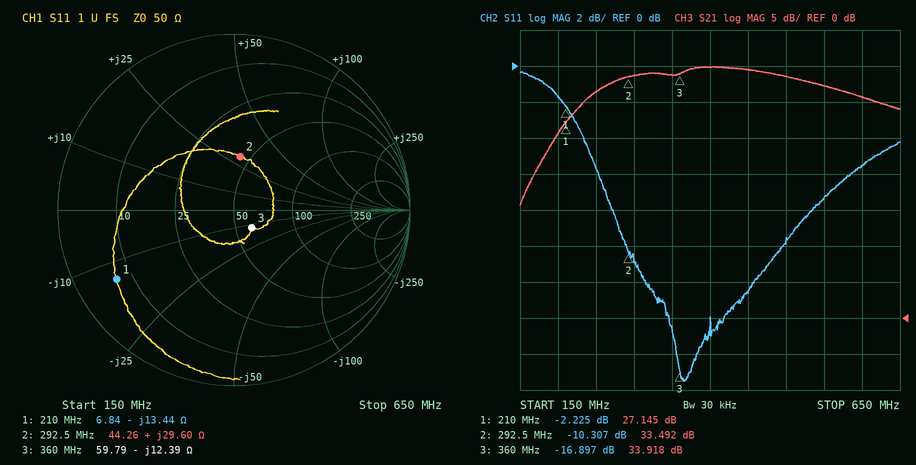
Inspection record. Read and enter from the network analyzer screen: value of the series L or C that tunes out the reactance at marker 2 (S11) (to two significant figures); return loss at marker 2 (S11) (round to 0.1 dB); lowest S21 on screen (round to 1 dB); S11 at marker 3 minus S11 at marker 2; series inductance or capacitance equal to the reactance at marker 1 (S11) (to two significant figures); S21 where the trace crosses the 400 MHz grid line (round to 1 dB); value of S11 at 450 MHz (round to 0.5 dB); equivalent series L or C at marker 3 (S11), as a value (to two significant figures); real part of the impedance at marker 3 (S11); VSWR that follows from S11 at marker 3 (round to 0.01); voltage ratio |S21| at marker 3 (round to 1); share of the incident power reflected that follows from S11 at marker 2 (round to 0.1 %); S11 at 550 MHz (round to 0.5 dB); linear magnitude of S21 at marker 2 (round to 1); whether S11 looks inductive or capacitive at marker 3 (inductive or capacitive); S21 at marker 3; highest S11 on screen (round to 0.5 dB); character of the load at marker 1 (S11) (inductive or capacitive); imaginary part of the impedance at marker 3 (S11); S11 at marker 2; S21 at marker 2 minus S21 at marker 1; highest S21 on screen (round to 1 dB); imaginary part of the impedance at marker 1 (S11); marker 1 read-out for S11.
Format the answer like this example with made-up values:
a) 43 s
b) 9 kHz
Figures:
a) 18 pF
b) 10.3 dB
c) 16 dB
d) -6.590 dB
e) 56 pF
f) 35 dB
g) -12.5 dB
h) 36 pF
i) 59.79 Ω
j) 1.33
k) 50
l) 9.3 %
m) -7.5 dB
n) 47
o) capacitive
p) 33.918 dB
q) -0.5 dB
r) capacitive
s) -12.39 Ω
t) -10.307 dB
u) 6.347 dB
v) 35 dB
w) -13.44 Ω
x) -2.225 dB
